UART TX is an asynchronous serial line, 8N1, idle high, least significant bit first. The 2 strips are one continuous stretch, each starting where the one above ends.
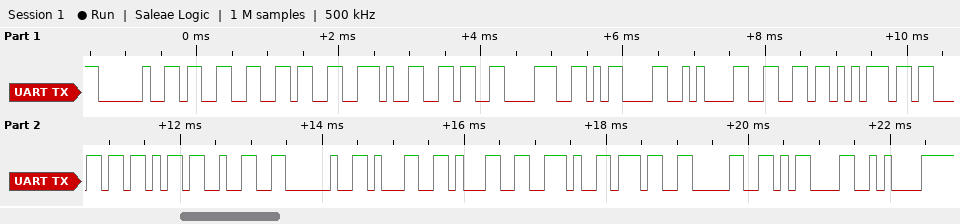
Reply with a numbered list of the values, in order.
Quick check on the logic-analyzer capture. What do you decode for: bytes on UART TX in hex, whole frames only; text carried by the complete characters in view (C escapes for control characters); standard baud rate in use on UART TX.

1. 0x20 0x33 0x36 0x2E 0x36 0x38 0x0D 0x0A 0x66 0x75 0x63 0x6B 0x32 0x20 0x31 0x31 0x2E 0x37 0x30 0x0D 0x0A
2. " 36.68\r\nfuck2 11.70\r\n"
3. 9600 baud
